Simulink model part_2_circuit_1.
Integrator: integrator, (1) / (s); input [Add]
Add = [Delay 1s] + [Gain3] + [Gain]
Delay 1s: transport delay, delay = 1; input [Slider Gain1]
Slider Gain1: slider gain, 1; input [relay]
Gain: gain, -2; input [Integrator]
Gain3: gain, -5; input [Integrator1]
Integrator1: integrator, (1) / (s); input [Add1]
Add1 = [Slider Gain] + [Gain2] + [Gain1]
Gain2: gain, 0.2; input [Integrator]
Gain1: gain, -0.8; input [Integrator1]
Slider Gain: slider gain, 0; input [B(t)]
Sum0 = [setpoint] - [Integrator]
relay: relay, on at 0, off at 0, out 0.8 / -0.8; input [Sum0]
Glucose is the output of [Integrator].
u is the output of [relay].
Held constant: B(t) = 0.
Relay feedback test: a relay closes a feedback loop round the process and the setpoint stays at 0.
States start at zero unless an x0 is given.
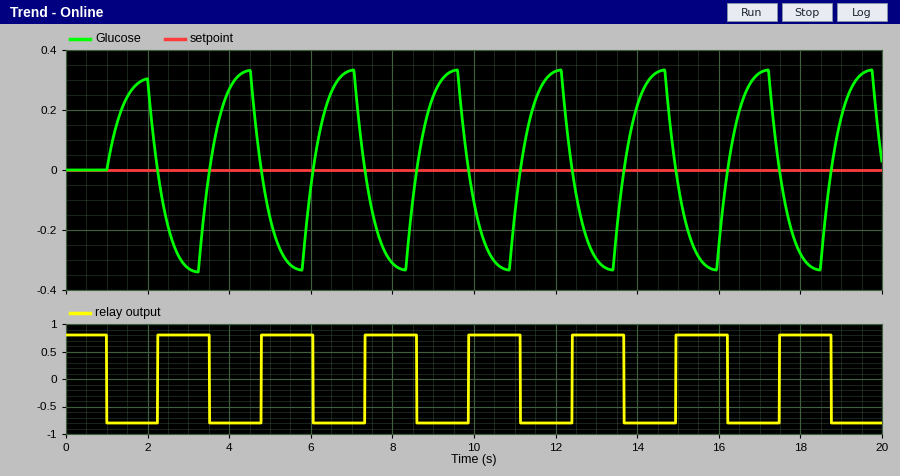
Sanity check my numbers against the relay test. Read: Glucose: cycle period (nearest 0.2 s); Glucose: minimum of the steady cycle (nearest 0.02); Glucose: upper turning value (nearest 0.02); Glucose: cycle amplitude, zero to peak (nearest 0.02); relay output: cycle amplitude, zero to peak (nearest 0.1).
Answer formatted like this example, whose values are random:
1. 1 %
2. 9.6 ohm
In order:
1. 2.6 s
2. -0.34
3. 0.34
4. 0.34
5. 0.8
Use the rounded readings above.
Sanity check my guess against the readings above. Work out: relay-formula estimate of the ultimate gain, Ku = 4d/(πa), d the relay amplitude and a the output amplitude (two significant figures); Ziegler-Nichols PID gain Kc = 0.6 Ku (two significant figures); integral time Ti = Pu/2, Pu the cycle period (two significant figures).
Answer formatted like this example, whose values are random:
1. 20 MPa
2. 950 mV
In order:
1. 3.0
2. 1.8
3. 1.3 s
